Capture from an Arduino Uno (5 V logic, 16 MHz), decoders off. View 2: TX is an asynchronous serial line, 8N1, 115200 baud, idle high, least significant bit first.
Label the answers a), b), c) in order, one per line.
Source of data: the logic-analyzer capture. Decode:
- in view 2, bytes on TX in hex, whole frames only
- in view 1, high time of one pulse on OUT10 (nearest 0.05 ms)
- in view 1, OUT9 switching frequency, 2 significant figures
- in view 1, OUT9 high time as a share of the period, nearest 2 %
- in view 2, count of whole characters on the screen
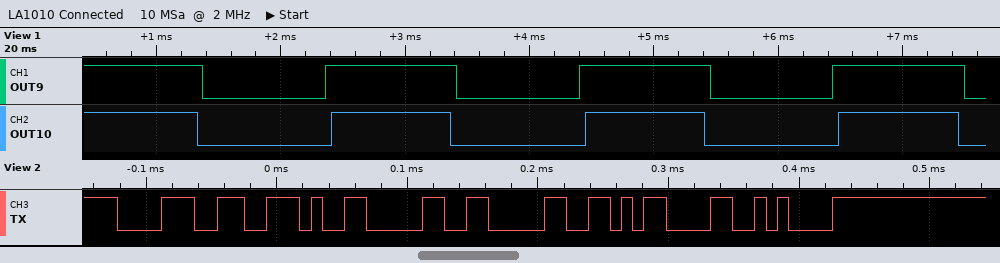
a) 38 2E 30 30 0D 0A
b) 0.95 ms
c) 490 Hz
d) 52 %
e) 6
